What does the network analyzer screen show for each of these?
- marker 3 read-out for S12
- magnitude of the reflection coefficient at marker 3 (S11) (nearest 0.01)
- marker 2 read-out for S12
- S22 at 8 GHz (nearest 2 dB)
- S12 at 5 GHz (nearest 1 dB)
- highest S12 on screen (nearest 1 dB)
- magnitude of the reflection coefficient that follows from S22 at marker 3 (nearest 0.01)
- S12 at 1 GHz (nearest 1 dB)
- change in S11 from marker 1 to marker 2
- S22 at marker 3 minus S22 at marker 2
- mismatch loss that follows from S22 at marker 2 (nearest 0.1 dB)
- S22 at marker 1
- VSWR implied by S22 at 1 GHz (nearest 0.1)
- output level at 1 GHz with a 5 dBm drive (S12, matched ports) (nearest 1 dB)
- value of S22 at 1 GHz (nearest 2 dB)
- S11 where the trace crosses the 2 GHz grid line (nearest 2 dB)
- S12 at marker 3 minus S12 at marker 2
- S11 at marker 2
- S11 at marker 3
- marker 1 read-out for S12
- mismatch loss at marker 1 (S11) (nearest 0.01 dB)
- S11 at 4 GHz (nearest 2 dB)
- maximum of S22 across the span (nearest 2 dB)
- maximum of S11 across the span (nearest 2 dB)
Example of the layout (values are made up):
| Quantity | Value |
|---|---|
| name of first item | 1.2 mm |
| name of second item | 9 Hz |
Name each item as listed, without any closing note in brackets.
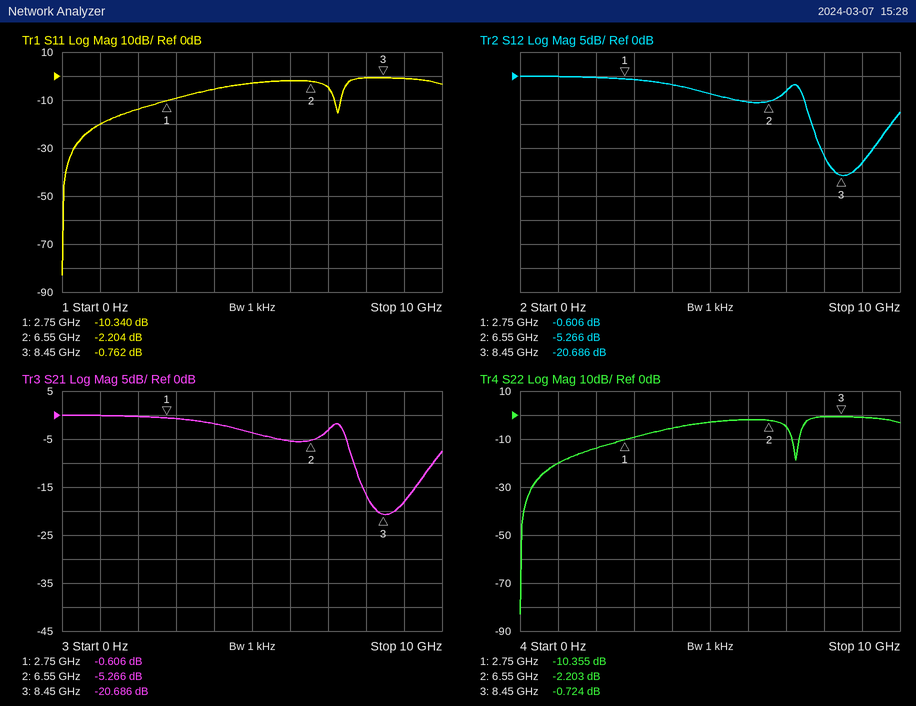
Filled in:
| Quantity | Value |
|---|---|
| marker 3 read-out for S12 | -20.686 dB |
| magnitude of the reflection coefficient at marker 3 (S11) | 0.92 |
| marker 2 read-out for S12 | -5.266 dB |
| S22 at 8 GHz | 0 dB |
| S12 at 5 GHz | -4 dB |
| highest S12 on screen | 0 dB |
| magnitude of the reflection coefficient that follows from S22 at marker 3 | 0.92 |
| S12 at 1 GHz | 0 dB |
| change in S11 from marker 1 to marker 2 | 8.136 dB |
| S22 at marker 3 minus S22 at marker 2 | 1.479 dB |
| mismatch loss that follows from S22 at marker 2 | 4.0 dB |
| S22 at marker 1 | -10.355 dB |
| VSWR implied by S22 at 1 GHz | 1.2 |
| output level at 1 GHz with a 5 dBm drive (S12, matched ports) | 5 dBm |
| value of S22 at 1 GHz | -20 dB |
| S11 where the trace crosses the 2 GHz grid line | -14 dB |
| S12 at marker 3 minus S12 at marker 2 | -15.420 dB |
| S11 at marker 2 | -2.204 dB |
| S11 at marker 3 | -0.762 dB |
| marker 1 read-out for S12 | -0.606 dB |
| mismatch loss at marker 1 (S11) | 0.42 dB |
| S11 at 4 GHz | -6 dB |
| maximum of S22 across the span | 0 dB |
| maximum of S11 across the span | 0 dB |
